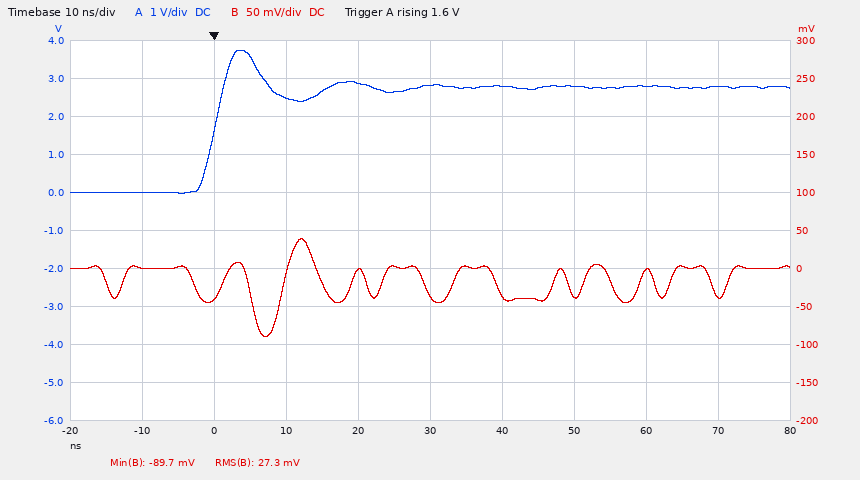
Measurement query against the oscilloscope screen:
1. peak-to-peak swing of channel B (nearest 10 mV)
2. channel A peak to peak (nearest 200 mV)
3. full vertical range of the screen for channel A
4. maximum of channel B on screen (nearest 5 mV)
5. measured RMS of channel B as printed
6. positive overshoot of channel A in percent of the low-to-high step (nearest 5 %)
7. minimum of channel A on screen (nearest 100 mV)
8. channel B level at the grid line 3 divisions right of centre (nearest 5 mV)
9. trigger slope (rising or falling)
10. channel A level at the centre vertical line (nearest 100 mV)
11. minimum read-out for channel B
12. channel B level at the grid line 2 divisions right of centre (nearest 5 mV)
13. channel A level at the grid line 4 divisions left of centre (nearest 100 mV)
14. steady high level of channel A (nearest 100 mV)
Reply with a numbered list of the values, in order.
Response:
1. 130 mV
2. 3.8 V
3. 10 V
4. 40 mV
5. 27.3 mV
6. 35 %
7. 0.0 V
8. -5 mV
9. rising
10. 2.8 V
11. -89.7 mV
12. -35 mV
13. 0.0 V
14. 2.8 V
